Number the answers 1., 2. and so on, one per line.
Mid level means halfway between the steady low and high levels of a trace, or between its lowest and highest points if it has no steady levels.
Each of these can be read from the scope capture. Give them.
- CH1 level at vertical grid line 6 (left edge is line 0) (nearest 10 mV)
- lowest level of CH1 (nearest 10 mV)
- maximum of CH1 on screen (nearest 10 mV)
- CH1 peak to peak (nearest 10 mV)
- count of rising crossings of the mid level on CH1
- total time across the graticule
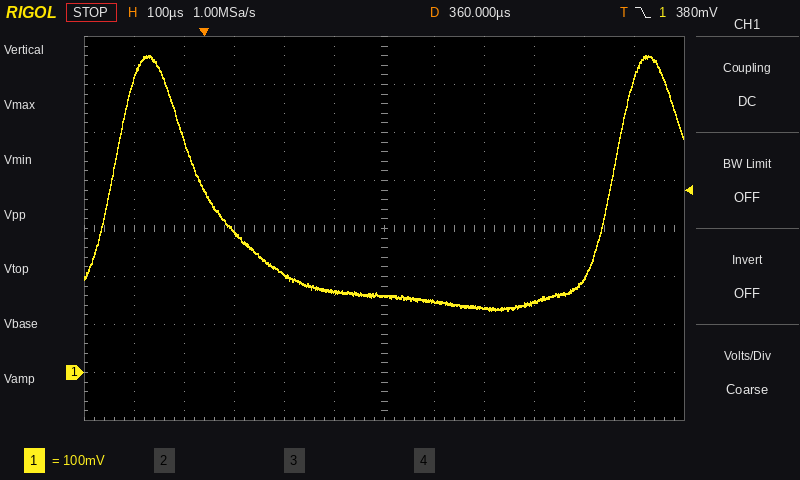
1. 160 mV
2. 130 mV
3. 660 mV
4. 530 mV
5. 2
6. 1.2 ms
